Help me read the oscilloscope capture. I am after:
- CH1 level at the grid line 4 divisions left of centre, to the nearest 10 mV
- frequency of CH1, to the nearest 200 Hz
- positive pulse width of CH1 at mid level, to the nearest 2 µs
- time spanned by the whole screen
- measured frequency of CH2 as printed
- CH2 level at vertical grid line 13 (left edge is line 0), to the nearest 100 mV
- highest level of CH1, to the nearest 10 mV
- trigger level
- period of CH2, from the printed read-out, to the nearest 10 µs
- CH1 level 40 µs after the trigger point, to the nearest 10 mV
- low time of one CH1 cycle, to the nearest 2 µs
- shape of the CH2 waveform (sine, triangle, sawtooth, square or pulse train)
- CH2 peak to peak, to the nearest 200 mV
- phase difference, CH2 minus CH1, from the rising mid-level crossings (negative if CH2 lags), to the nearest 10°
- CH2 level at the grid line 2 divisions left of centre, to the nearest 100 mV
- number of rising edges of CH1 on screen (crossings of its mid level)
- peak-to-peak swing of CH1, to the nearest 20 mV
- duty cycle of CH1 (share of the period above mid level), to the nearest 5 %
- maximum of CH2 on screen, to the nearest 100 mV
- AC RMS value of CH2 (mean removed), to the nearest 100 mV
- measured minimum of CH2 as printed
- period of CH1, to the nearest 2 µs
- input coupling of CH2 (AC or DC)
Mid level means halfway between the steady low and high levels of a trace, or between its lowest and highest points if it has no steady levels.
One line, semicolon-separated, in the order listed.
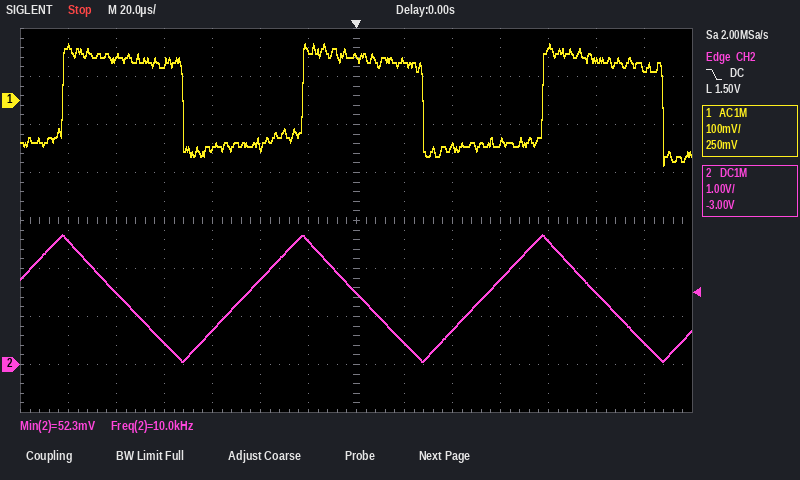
80 mV; 10.0 kHz; 50 µs; 280 µs; 10.0 kHz; 500 mV; 120 mV; 1.50 V; 100 µs; -90 mV; 50 µs; triangle; 2.6 V; +90°; 1.8 V; 3; 260 mV; 50 %; 2.7 V; 800 mV; 52.3 mV; 100 µs; DC
